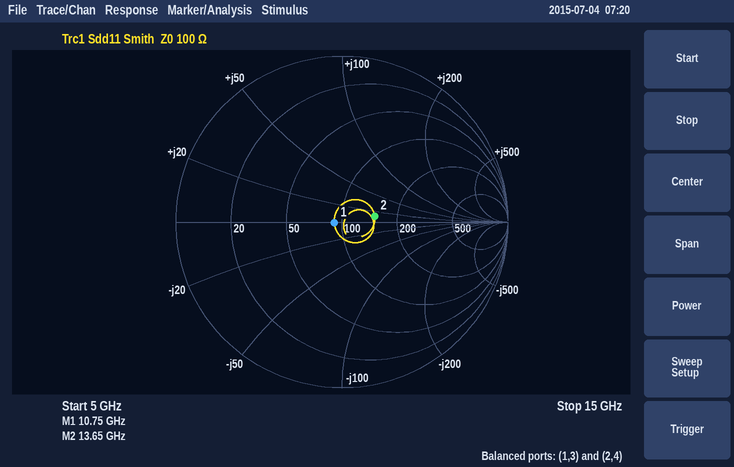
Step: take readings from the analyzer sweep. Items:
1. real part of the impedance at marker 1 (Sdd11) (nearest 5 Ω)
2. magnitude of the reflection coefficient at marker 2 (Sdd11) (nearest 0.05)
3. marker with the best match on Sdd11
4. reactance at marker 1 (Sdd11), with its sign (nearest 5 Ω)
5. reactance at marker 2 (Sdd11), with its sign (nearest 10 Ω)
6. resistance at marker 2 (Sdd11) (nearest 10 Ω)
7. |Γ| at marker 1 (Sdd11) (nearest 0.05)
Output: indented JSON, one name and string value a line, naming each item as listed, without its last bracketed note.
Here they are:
{
  "real part of the impedance at marker 1 (Sdd11)": "90 Ω",
  "magnitude of the reflection coefficient at marker 2 (Sdd11)": "0.20",
  "marker with the best match on Sdd11": "marker 1",
  "reactance at marker 1 (Sdd11), with its sign": "0 Ω",
  "reactance at marker 2 (Sdd11), with its sign": "+10 Ω",
  "resistance at marker 2 (Sdd11)": "150 Ω",
  "|Γ| at marker 1 (Sdd11)": "0.05"
}
